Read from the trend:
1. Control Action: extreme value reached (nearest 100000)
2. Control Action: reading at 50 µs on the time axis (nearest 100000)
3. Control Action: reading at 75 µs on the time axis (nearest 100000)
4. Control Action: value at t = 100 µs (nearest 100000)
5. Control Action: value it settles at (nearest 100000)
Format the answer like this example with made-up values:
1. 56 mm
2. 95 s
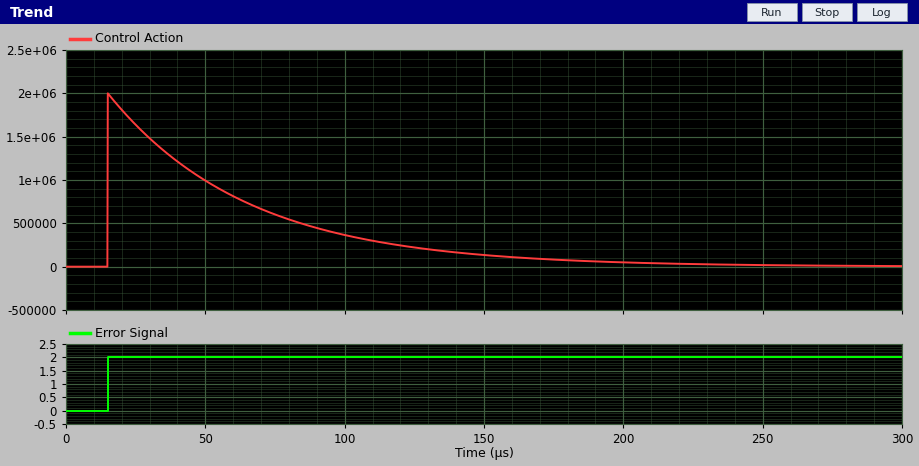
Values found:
1. 2000000
2. 1000000
3. 600000
4. 400000
5. 0
